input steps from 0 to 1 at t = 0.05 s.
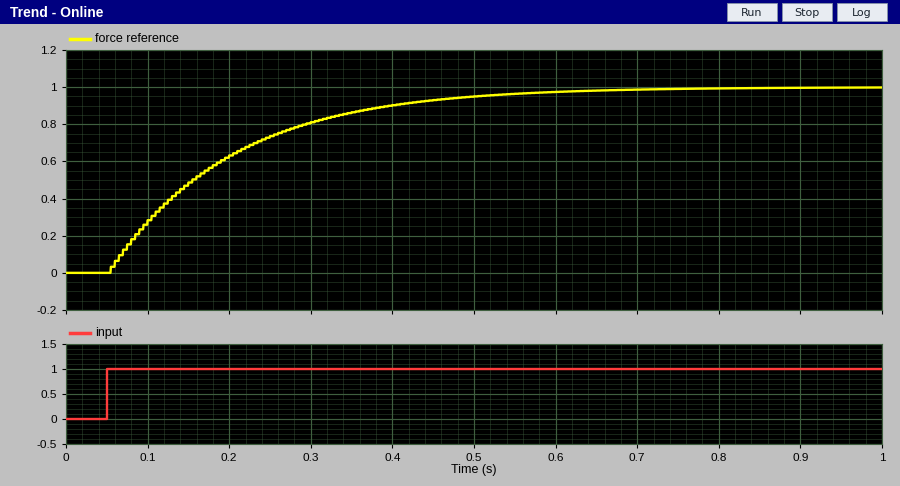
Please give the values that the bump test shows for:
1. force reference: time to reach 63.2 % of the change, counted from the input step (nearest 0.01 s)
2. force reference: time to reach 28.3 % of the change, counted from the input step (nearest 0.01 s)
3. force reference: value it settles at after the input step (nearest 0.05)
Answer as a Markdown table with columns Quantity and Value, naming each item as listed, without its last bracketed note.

| Quantity | Value |
|---|---|
| force reference: time to reach 63.2 % of the change, counted from the input step | 0.15 s |
| force reference: time to reach 28.3 % of the change, counted from the input step | 0.05 s |
| force reference: value it settles at after the input step | 1.00 |
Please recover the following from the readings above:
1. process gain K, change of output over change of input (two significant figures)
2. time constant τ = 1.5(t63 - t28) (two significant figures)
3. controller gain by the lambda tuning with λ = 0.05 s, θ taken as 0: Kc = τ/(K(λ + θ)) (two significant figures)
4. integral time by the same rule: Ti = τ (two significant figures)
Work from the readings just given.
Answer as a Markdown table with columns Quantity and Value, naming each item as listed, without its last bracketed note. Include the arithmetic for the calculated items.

| Quantity | Value |
|---|---|
| process gain K, change of output over change of input | (1 - 0) / 1 = 1.0 |
| time constant τ = 1.5(t63 - t28) | 1.5 × (0.15 - 0.05) = 0.15 s |
| controller gain by the lambda tuning with λ = 0.05 s, θ taken as 0: Kc = τ/(K(λ + θ)) | 0.15 / (1 × (0.05 + 0)) = 3.0 |
| integral time by the same rule: Ti = τ | 0.15 s |
